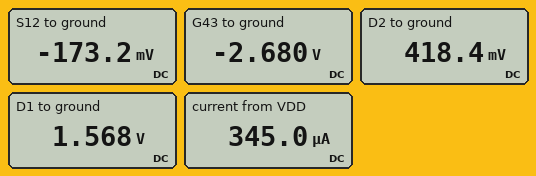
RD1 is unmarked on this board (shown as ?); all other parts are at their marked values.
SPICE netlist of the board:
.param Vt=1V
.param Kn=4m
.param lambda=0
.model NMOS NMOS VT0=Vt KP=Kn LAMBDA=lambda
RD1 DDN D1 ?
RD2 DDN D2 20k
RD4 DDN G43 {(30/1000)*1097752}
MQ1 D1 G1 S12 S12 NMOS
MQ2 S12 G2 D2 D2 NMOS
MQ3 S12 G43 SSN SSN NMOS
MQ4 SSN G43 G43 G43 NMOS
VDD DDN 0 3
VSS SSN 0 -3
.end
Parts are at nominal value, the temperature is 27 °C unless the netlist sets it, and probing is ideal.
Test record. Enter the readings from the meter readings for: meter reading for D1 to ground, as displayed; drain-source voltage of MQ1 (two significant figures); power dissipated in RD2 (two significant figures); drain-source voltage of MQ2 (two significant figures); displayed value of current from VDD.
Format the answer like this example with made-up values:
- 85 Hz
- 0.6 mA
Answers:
- 1.568 V
- 1.7 V
- 330 µW
- -590 mV
- 345.0 µA
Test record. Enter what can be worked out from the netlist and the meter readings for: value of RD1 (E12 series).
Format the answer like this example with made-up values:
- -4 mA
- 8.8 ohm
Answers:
- 33 kΩ
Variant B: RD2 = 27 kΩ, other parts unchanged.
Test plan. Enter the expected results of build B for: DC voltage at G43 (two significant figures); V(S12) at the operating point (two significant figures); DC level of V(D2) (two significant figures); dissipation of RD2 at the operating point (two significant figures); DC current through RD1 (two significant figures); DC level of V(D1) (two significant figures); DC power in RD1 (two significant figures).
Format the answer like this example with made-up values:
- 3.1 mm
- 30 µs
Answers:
- -2.7 V
- -220 mV
- 340 mV
- 260 µW
- 74 µA
- 560 mV
- 180 µW
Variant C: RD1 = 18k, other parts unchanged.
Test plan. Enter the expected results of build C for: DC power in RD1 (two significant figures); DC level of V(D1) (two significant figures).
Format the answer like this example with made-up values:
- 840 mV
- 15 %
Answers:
- 34 µW
- 2.2 V
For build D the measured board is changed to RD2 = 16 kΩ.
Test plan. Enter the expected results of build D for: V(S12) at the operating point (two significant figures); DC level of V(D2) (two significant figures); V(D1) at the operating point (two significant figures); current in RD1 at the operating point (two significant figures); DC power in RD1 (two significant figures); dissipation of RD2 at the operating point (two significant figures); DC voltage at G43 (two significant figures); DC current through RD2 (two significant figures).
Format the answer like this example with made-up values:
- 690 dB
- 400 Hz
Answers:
- -110 mV
- 490 mV
- 2.5 V
- 16 µA
- 8.1 µW
- 390 µW
- -2.7 V
- 160 µA
